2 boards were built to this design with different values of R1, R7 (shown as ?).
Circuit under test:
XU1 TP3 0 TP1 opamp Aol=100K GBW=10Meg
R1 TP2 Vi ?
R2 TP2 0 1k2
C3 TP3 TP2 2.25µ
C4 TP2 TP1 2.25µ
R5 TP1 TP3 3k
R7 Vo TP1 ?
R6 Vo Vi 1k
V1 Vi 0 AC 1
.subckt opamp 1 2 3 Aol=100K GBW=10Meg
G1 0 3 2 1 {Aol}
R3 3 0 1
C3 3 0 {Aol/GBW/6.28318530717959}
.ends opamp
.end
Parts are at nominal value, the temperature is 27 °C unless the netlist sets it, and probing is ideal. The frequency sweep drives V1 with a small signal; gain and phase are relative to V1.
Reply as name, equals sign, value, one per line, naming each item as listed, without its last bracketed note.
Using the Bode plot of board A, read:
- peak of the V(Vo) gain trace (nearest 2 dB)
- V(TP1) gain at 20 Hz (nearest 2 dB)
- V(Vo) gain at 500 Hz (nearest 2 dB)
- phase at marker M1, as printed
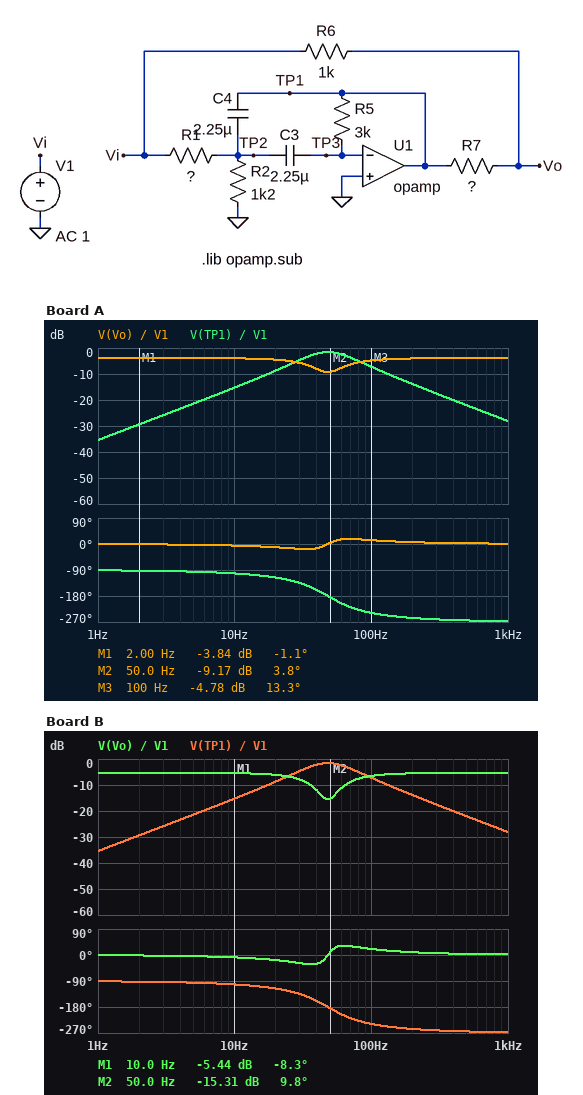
peak of the V(Vo) gain trace = -4 dB
V(TP1) gain at 20 Hz = -8 dB
V(Vo) gain at 500 Hz = -4 dB
phase at marker M1, as printed = -1.1 deg
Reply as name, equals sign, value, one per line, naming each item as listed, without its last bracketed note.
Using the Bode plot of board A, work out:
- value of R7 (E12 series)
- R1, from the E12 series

value of R7 = 1.8 kΩ
R1, from the E12 series = 1.8 kΩ
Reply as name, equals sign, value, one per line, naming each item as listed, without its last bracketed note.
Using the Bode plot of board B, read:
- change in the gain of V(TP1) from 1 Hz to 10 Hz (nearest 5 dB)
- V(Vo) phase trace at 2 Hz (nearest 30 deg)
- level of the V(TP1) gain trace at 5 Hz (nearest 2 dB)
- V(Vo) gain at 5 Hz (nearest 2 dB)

change in the gain of V(TP1) from 1 Hz to 10 Hz = 20 dB
V(Vo) phase trace at 2 Hz = 0 deg
level of the V(TP1) gain trace at 5 Hz = -22 dB
V(Vo) gain at 5 Hz = -6 dB
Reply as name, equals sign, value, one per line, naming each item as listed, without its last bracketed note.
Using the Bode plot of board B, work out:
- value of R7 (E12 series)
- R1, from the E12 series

value of R7 = 1.2 kΩ
R1, from the E12 series = 1.8 kΩ
